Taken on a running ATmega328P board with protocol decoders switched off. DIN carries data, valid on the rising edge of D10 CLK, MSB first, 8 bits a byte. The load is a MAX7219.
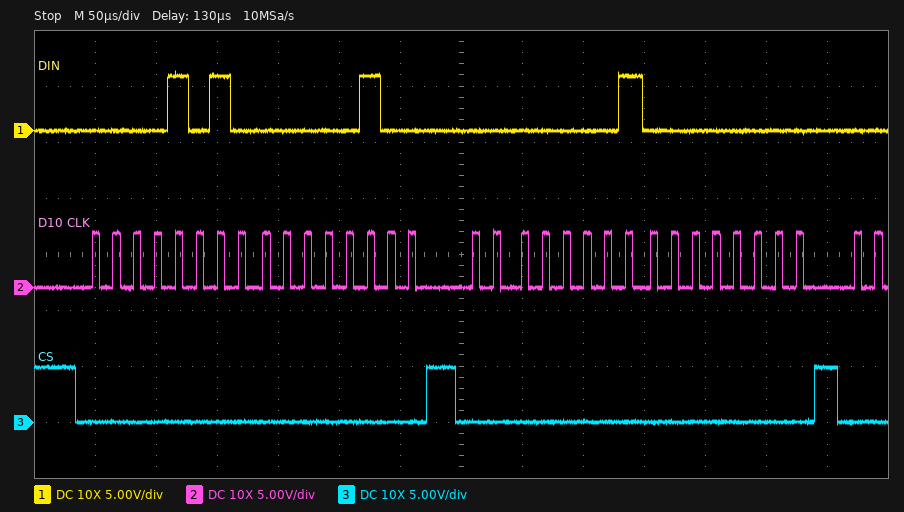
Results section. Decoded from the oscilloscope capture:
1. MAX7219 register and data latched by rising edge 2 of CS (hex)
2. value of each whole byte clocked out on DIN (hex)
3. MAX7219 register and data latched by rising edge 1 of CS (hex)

register 0x1, data 0x00
0x0A 0x04 0x01 0x00
register 0xA, data 0x04
